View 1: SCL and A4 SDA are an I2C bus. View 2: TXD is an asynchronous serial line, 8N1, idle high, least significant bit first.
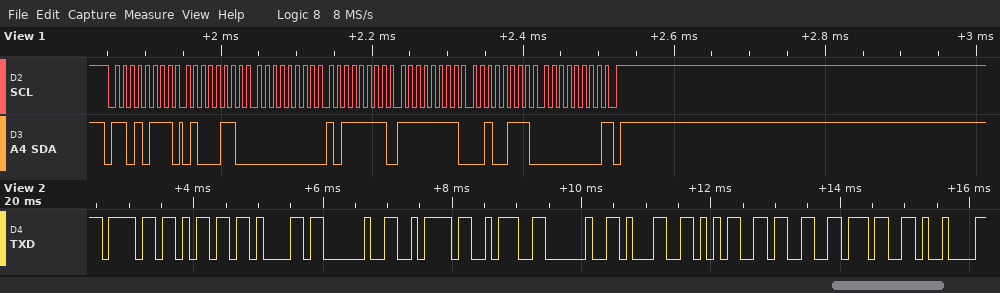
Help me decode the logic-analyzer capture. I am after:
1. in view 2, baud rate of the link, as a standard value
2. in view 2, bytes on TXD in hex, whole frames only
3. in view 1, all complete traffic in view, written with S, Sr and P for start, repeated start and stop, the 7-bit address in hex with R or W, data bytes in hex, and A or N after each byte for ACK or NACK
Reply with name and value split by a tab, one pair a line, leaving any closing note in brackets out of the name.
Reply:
in view 2, baud rate of the link, as a standard value	9600 baud
in view 2, bytes on TXD in hex, whole frames only	6F 6D 61 20 7A 3A 20 31 35 33 37 09
in view 1, all complete traffic in view, written with S, Sr and P for start, repeated start and stop, the 7-bit address in hex with R or W, data bytes in hex, and A or N after each byte for ACK or NACK	S 6BR A 46 A 00 A BF A FF A 27 A 00 N P
